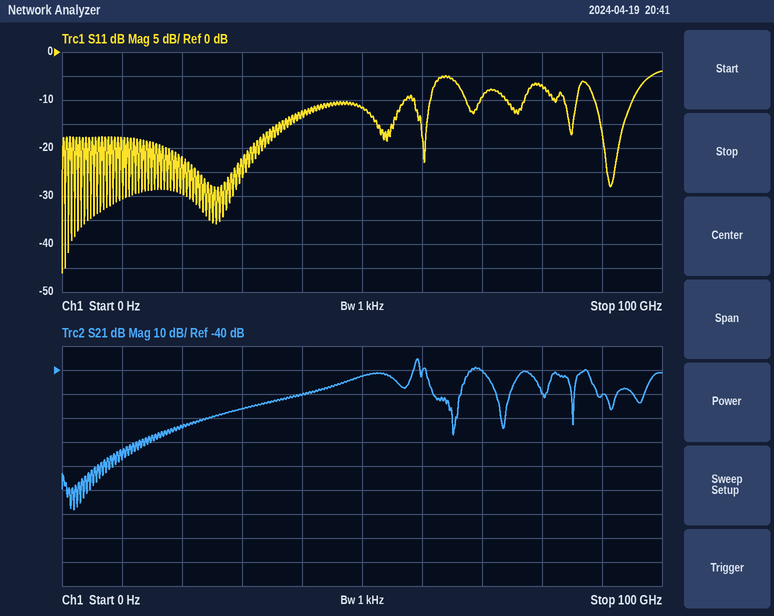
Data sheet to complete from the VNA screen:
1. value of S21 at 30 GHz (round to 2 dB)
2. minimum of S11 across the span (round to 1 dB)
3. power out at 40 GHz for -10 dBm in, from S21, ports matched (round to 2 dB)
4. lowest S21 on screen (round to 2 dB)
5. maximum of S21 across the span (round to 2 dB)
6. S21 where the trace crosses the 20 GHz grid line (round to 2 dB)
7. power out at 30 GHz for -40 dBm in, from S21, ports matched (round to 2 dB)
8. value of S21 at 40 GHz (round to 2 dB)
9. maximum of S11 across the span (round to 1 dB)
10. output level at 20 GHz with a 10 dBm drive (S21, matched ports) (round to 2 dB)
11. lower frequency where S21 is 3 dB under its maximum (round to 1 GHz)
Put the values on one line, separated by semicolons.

-56 dB; -46 dB; -60 dBm; -98 dB; -36 dB; -64 dB; -96 dBm; -50 dB; -4 dB; -54 dBm; 59 GHz
